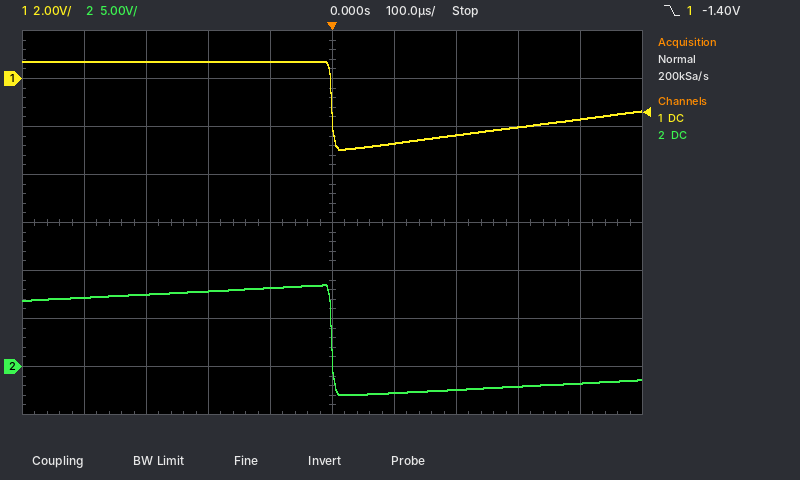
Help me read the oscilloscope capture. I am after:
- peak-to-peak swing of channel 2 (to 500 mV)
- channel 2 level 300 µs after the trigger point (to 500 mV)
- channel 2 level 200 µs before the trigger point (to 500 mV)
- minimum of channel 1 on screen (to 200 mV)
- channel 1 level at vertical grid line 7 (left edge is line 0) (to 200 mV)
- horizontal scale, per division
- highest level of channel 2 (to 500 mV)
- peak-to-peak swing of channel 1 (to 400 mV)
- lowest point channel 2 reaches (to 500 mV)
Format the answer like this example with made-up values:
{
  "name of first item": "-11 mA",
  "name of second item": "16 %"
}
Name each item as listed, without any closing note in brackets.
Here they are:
{
  "peak-to-peak swing of channel 2": "11.5 V",
  "channel 2 level 300 µs after the trigger point": "-2.0 V",
  "channel 2 level 200 µs before the trigger point": "8.0 V",
  "minimum of channel 1 on screen": "-3.0 V",
  "channel 1 level at vertical grid line 7 (left edge is line 0)": "-2.4 V",
  "horizontal scale, per division": "100 µs",
  "highest level of channel 2": "8.5 V",
  "peak-to-peak swing of channel 1": "3.6 V",
  "lowest point channel 2 reaches": "-3.0 V"
}
